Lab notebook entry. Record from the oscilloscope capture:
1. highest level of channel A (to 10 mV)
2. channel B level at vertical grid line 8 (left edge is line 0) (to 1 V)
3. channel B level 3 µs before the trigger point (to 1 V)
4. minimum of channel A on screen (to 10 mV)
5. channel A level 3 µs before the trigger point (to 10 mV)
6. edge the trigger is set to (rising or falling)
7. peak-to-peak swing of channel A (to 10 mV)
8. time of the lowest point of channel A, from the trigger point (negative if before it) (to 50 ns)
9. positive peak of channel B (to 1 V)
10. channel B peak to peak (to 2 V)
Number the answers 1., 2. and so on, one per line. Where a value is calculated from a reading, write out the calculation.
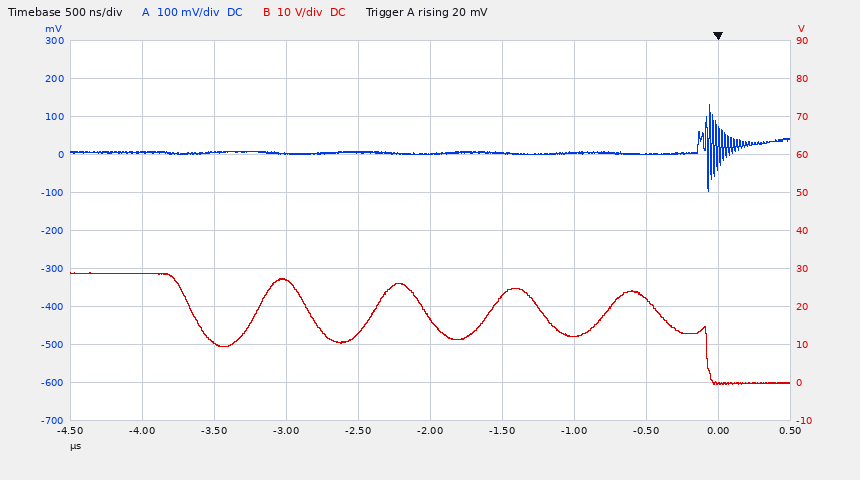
1. 130 mV
2. 22 V
3. 27 V
4. -100 mV
5. 0 mV
6. rising
7. 130 mV − (-100 mV) = 230 mV
8. -50 ns
9. 29 V
10. 30 V
